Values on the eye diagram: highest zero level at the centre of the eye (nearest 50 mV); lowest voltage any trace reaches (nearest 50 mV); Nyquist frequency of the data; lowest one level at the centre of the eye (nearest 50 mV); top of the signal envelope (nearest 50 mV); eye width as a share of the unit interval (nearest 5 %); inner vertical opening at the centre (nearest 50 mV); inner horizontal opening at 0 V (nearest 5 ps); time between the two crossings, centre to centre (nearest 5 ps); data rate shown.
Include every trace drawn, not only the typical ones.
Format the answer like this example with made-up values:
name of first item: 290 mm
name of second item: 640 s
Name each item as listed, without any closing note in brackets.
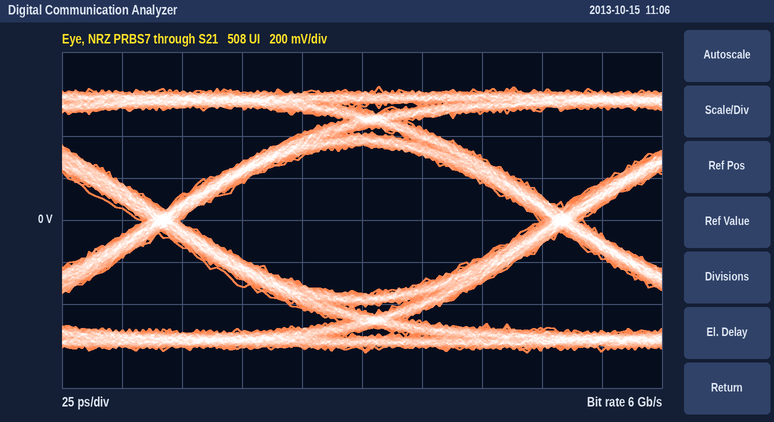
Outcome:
highest zero level at the centre of the eye: -350 mV
lowest voltage any trace reaches: -650 mV
Nyquist frequency of the data: 3 GHz
lowest one level at the centre of the eye: 350 mV
top of the signal envelope: 650 mV
eye width as a share of the unit interval: 90 %
inner vertical opening at the centre: 700 mV
inner horizontal opening at 0 V: 150 ps
time between the two crossings, centre to centre: 165 ps
data rate shown: 6 Gb/s
